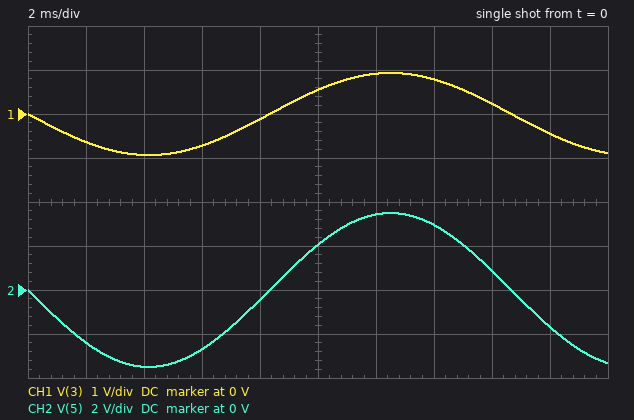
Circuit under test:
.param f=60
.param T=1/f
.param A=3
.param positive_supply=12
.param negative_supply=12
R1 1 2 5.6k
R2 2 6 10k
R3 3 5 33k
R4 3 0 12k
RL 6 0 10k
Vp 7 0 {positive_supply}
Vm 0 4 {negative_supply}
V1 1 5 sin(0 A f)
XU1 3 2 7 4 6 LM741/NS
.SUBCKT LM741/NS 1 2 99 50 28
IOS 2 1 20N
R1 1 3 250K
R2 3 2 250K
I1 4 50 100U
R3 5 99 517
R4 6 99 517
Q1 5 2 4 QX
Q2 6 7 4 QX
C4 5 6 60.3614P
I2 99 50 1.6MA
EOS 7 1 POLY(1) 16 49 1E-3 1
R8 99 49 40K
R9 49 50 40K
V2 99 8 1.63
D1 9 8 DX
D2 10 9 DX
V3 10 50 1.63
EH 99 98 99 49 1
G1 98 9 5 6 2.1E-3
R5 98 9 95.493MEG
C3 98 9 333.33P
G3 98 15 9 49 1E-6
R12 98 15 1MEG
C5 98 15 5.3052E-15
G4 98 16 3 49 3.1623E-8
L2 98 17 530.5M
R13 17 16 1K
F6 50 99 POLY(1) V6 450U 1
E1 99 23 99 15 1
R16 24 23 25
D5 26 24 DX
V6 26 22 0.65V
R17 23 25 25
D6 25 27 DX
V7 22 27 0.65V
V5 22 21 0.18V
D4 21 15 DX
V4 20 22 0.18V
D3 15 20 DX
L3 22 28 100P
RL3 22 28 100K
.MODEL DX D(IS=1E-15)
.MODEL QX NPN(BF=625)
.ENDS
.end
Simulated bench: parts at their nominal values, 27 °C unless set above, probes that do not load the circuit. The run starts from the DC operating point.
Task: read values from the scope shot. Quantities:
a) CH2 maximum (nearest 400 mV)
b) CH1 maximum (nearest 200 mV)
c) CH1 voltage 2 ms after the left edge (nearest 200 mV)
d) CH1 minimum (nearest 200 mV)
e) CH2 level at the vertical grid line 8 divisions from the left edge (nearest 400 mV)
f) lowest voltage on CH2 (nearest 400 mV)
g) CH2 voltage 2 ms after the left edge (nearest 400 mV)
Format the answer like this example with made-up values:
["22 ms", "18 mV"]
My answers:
["3.6 V", "1.0 V", "-600 mV", "-1.0 V", "800 mV", "-3.6 V", "-2.4 V"]
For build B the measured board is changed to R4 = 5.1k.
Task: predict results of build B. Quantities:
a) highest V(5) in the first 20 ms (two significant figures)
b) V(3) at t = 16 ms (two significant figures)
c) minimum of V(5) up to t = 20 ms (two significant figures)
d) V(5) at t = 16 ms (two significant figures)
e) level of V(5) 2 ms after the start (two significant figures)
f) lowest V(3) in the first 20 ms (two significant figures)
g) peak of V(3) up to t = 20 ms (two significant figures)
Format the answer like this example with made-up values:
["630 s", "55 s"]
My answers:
["3.0 V", "98 mV", "-3.0 V", "740 mV", "-2.0 V", "-400 mV", "400 mV"]
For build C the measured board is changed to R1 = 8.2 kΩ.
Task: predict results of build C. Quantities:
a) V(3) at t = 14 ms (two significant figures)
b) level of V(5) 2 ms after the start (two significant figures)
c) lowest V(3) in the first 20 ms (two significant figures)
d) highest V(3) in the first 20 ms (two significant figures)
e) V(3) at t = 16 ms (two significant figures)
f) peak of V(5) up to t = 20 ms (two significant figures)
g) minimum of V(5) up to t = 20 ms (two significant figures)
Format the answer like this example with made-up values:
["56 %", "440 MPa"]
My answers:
["740 mV", "-2.2 V", "-870 mV", "870 mV", "220 mV", "3.3 V", "-3.3 V"]
